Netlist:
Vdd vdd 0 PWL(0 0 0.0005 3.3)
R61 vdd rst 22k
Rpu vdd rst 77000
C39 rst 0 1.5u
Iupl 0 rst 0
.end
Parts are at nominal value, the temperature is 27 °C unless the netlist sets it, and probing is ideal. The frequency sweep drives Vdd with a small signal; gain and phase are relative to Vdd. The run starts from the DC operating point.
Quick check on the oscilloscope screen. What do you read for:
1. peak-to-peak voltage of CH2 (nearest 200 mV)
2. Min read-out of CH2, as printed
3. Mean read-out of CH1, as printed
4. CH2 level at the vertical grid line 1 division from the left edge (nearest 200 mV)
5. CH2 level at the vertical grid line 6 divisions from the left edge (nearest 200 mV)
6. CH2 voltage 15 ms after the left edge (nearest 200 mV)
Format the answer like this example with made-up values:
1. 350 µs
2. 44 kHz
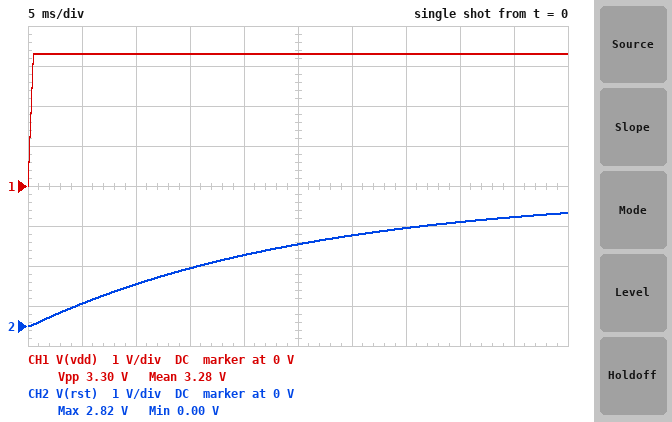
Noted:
1. 2.8 V
2. 0.00 V
3. 3.28 V
4. 600 mV
5. 2.2 V
6. 1.4 V
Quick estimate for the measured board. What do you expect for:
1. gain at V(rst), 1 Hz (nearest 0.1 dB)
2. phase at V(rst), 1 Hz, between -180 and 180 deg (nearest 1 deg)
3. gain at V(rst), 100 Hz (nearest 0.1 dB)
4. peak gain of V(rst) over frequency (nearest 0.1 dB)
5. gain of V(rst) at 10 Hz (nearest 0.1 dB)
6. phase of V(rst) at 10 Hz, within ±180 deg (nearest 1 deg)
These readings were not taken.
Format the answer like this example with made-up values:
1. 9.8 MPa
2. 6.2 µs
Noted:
1. -0.1 dB
2. -9 deg
3. -24.2 dB
4. 0 dB
5. -5.6 dB
6. -58 deg
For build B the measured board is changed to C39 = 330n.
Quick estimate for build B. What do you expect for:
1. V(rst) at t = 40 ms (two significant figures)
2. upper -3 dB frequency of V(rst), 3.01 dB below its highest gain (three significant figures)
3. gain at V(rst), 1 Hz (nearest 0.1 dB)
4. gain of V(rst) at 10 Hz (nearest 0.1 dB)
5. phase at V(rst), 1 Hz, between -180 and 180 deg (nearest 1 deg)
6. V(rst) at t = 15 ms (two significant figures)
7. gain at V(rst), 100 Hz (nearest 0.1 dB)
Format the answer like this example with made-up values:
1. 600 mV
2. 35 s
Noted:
1. 3.3 V
2. 28.2 Hz
3. 0 dB
4. -0.5 dB
5. -2 deg
6. 3.1 V
7. -11.3 dB
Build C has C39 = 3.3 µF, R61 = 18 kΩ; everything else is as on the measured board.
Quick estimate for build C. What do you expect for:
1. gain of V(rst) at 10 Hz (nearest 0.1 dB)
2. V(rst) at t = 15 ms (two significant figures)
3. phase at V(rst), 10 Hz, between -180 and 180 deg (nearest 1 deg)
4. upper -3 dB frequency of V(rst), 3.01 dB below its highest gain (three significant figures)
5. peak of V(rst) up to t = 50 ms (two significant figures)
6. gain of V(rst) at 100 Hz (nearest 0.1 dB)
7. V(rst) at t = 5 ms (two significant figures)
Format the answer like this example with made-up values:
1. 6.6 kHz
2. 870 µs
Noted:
1. -10.1 dB
2. 870 mV
3. -72 deg
4. 3.31 Hz
5. 2.1 V
6. -29.6 dB
7. 310 mV
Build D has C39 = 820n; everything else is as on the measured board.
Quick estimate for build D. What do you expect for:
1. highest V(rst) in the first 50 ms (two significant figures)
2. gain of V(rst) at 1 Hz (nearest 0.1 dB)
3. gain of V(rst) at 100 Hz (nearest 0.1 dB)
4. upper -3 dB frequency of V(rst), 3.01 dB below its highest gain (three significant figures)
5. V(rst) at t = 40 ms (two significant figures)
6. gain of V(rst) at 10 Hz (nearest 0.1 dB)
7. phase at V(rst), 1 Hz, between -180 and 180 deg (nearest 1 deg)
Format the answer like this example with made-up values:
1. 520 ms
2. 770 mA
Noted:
1. 3.2 V
2. 0 dB
3. -19.0 dB
4. 11.3 Hz
5. 3.1 V
6. -2.5 dB
7. -5 deg
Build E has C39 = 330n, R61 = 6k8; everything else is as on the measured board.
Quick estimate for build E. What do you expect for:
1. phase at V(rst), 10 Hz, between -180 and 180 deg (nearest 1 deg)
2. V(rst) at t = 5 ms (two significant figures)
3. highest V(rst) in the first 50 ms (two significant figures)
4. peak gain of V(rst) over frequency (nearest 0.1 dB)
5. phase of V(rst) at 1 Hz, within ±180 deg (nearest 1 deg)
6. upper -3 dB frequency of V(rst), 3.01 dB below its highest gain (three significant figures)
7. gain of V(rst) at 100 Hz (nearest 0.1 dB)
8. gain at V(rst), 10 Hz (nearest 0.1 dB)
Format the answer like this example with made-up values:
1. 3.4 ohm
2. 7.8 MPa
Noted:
1. -7 deg
2. 3.0 V
3. 3.3 V
4. 0 dB
5. -1 deg
6. 77.2 Hz
7. -4.3 dB
8. -0.1 dB
